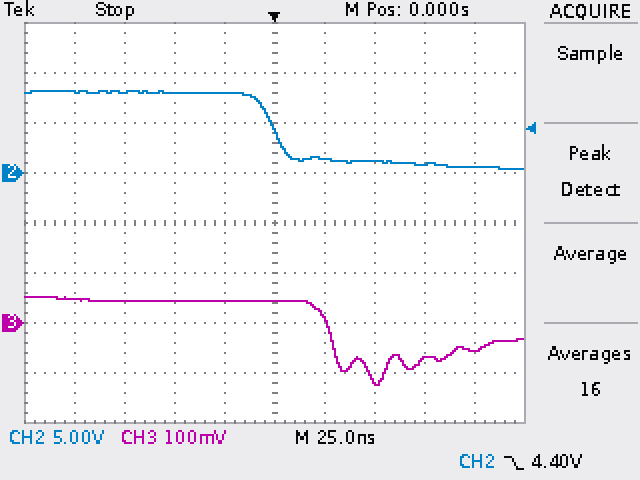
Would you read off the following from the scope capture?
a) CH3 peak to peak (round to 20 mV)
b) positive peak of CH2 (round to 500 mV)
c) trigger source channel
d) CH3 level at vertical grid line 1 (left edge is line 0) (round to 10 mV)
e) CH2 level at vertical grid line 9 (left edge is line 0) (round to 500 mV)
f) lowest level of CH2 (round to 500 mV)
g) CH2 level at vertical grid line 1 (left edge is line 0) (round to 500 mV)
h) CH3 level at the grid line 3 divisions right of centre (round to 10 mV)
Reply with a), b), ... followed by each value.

a) 180 mV
b) 8.0 V
c) CH2
d) 50 mV
e) 500 mV
f) 500 mV
g) 8.0 V
h) -70 mV
